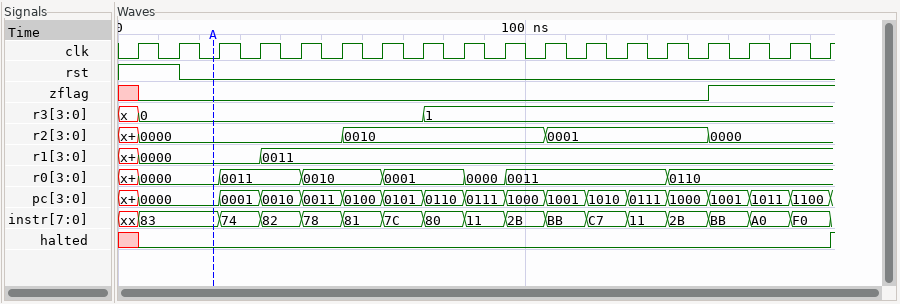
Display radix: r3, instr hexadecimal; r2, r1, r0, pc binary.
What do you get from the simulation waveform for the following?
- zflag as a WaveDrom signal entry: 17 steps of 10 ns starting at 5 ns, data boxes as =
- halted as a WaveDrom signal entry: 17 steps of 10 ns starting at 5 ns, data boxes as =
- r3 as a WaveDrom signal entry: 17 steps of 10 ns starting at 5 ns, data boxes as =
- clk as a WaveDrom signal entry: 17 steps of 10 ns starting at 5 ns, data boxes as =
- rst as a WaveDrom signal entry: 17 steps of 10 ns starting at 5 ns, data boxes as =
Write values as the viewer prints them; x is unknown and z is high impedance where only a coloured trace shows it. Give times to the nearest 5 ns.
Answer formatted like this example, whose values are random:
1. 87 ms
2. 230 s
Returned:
1. {name: 'zflag', wave: '0.............1..'}
2. {name: 'halted', wave: '0................'}
3. {name: 'r3', wave: '=......=.........', data: '0 1'}
4. {name: 'clk', wave: 'p................'}
5. {name: 'rst', wave: '10...............'}
